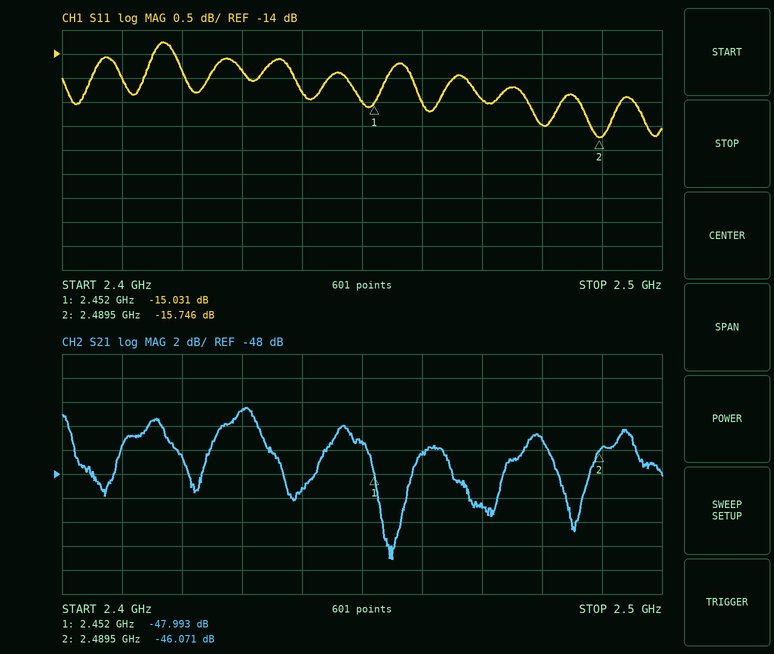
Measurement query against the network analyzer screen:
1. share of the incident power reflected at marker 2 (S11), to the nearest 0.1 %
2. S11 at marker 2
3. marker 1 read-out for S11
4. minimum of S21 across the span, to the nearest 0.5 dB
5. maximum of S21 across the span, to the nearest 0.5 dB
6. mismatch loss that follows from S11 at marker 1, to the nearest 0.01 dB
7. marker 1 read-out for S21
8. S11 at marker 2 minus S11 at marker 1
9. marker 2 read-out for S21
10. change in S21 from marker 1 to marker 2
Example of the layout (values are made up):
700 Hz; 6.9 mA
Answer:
2.7 %; -15.746 dB; -15.031 dB; -55.0 dB; -42.5 dB; 0.14 dB; -47.993 dB; -0.715 dB; -46.071 dB; 1.922 dB
